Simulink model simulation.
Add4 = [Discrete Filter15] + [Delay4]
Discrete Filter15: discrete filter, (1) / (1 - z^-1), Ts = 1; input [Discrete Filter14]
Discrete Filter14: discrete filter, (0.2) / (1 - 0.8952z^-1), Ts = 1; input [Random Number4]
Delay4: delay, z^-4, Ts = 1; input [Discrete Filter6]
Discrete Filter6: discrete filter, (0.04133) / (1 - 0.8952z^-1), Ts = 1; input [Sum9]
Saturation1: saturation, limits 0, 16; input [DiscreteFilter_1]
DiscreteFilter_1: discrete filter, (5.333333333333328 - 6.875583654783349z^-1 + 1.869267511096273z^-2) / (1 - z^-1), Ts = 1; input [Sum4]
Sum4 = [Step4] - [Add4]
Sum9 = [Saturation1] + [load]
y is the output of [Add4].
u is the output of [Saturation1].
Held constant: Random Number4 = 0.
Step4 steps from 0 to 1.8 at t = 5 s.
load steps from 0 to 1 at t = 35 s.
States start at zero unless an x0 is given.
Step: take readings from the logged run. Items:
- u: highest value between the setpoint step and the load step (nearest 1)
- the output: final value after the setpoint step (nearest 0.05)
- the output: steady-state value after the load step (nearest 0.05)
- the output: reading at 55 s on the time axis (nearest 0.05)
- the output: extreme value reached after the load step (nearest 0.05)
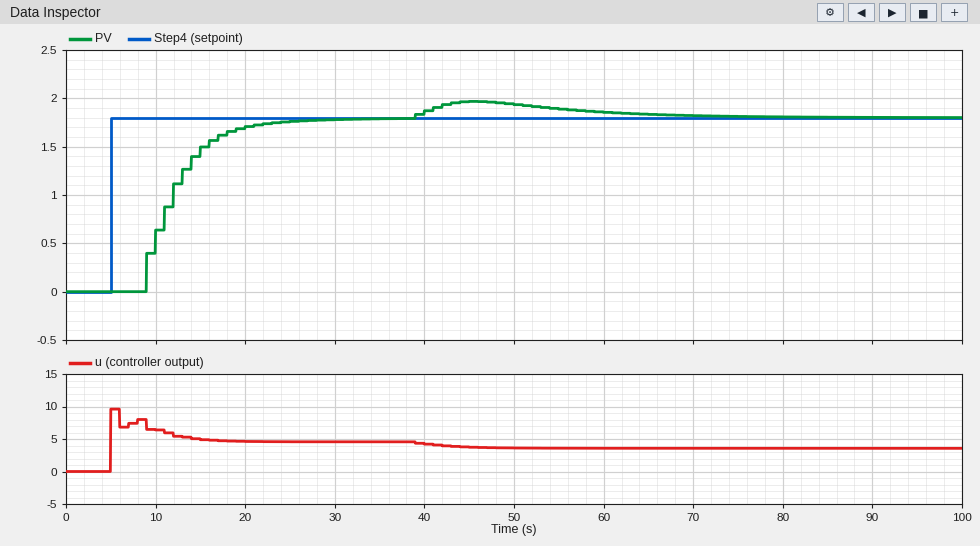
10
1.80
1.80
1.90
1.95
